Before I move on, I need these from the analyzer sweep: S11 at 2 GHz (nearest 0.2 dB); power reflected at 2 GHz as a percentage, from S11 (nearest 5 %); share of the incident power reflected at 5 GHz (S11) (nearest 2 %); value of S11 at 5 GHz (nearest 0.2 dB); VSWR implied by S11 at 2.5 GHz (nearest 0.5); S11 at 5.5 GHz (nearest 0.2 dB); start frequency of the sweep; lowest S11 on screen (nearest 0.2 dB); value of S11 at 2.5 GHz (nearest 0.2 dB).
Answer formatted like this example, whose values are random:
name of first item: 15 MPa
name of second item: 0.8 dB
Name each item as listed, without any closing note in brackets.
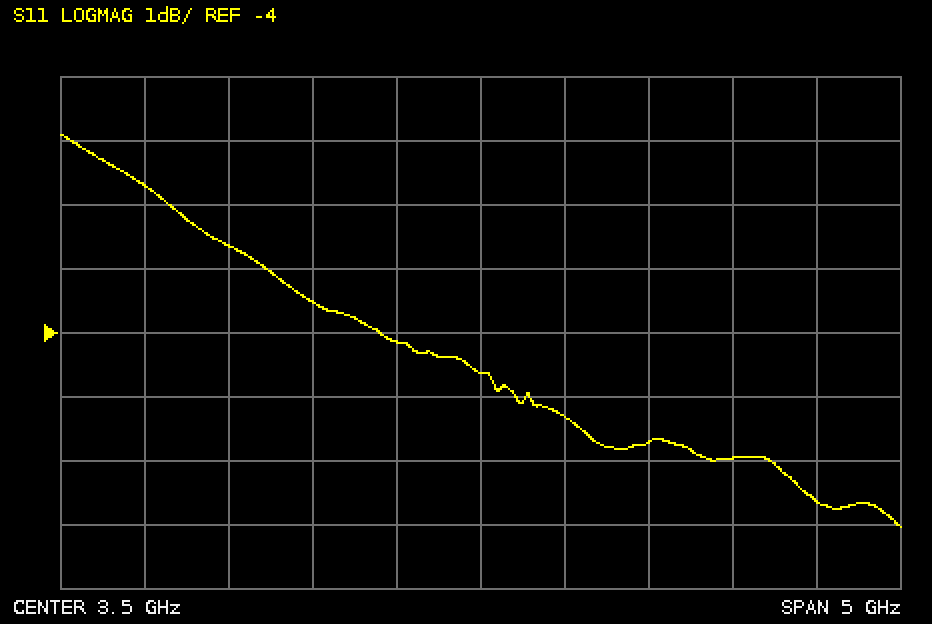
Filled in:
S11 at 2 GHz: -2.6 dB
power reflected at 2 GHz as a percentage, from S11: 55 %
share of the incident power reflected at 5 GHz (S11): 26 %
value of S11 at 5 GHz: -6.0 dB
VSWR implied by S11 at 2.5 GHz: 5.0
S11 at 5.5 GHz: -6.6 dB
start frequency of the sweep: 1 GHz
lowest S11 on screen: -7.0 dB
value of S11 at 2.5 GHz: -3.6 dB
